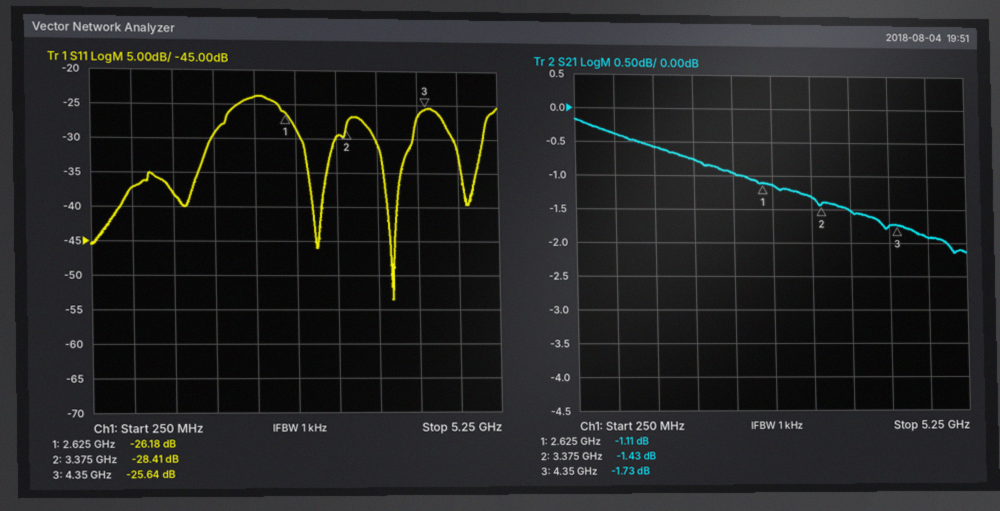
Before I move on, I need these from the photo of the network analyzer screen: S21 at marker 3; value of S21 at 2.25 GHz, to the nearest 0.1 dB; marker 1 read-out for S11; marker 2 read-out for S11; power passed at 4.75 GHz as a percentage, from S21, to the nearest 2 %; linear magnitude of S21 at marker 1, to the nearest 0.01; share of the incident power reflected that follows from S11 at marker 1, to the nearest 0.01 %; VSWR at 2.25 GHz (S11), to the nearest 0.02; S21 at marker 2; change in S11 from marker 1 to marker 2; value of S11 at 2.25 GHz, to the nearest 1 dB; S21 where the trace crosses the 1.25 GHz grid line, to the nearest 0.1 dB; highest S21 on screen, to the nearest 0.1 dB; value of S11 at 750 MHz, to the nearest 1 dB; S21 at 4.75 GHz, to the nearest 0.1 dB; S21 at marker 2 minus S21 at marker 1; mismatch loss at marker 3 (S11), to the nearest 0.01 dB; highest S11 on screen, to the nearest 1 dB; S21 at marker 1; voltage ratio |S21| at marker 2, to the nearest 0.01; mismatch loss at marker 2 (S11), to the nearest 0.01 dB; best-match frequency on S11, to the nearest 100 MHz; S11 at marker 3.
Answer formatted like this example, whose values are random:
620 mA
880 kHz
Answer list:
-1.73 dB
-1.0 dB
-26.18 dB
-28.41 dB
64 %
0.88
0.24 %
1.14
-1.43 dB
-2.23 dB
-24 dB
-0.6 dB
-0.2 dB
-37 dB
-1.9 dB
-0.32 dB
0.01 dB
-24 dB
-1.11 dB
0.85
0.01 dB
3.9 GHz
-25.64 dB
